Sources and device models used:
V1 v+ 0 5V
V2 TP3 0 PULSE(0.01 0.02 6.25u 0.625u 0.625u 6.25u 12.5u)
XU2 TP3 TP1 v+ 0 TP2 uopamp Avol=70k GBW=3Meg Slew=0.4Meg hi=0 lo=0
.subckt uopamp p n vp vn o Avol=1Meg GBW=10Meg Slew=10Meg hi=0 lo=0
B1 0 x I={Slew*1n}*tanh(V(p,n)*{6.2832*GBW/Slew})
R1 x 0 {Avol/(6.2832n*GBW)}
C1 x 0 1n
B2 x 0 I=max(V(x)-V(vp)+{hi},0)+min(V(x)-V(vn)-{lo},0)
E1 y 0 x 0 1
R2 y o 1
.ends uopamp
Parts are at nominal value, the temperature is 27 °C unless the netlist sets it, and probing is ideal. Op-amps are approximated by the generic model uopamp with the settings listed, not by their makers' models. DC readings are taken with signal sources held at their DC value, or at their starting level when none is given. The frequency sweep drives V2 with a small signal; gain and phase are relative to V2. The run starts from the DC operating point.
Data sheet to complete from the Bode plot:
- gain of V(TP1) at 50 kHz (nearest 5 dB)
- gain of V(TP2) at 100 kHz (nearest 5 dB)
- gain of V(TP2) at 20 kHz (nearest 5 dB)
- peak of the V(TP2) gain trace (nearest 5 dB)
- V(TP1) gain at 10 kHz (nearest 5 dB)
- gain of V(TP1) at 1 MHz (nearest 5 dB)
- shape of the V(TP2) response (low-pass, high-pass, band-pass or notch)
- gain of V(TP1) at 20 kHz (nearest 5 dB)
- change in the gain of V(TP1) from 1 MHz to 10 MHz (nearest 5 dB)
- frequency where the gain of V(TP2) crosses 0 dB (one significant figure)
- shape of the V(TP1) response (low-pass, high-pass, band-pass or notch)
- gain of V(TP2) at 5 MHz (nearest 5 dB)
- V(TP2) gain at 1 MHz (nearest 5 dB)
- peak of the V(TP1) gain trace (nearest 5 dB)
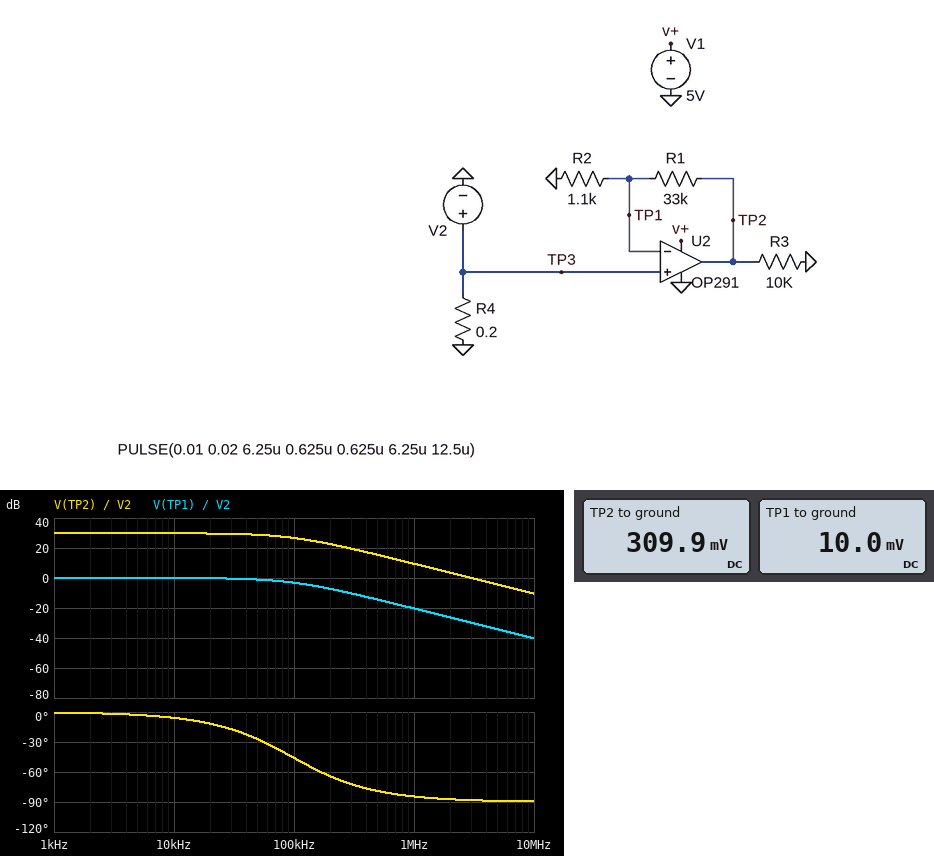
0 dB
25 dB
30 dB
30 dB
0 dB
-20 dB
low-pass
0 dB
-20 dB
3 MHz
low-pass
-5 dB
10 dB
0 dB
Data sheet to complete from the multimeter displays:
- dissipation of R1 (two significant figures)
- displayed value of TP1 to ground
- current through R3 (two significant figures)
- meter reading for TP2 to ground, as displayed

2.7 µW
10.0 mV
31 µA
309.9 mV
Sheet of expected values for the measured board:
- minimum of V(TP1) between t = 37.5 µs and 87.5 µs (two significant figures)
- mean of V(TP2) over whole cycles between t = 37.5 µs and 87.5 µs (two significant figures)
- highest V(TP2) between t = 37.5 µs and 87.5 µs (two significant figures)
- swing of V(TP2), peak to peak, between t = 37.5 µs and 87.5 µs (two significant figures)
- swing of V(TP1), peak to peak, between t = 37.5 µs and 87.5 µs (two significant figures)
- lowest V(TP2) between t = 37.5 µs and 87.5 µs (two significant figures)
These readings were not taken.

10 mV
480 mV
610 mV
290 mV
9.4 mV
320 mV
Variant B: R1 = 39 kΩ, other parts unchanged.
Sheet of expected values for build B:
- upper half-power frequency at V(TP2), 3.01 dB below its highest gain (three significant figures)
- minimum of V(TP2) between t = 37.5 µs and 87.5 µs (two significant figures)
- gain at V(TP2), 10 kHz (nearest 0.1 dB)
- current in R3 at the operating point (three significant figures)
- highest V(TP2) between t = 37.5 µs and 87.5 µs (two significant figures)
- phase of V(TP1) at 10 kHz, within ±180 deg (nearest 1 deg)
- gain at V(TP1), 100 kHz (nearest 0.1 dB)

82.3 kHz
390 mV
31.2 dB
36.4 µA
720 mV
-7 deg
-3.9 dB
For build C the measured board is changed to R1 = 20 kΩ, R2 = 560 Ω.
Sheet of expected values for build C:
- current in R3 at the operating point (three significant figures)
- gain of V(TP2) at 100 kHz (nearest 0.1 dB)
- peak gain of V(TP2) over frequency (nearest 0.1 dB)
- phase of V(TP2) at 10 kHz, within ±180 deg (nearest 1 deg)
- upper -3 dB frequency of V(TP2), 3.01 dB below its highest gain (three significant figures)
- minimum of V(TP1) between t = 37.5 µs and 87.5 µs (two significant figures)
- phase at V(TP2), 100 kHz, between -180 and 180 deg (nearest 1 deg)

36.7 µA
27.3 dB
31.3 dB
-7 deg
81.7 kHz
11 mV
-51 deg
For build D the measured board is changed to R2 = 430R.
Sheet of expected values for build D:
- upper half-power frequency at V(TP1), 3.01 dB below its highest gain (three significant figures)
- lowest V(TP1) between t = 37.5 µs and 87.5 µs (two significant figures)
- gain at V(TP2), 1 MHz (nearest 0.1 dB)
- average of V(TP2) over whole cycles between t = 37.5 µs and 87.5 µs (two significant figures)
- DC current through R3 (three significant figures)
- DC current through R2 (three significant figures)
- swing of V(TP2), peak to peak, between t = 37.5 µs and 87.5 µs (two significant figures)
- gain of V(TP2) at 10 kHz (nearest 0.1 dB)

38.6 kHz
12 mV
9.5 dB
1.2 V
77.7 µA
23.2 µA
470 mV
37.5 dB
